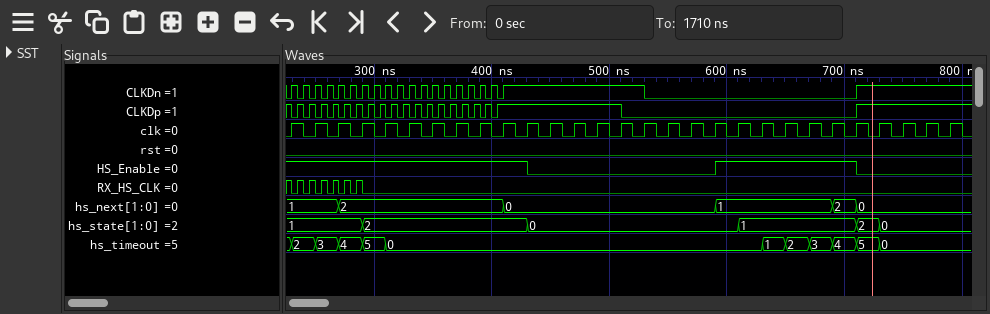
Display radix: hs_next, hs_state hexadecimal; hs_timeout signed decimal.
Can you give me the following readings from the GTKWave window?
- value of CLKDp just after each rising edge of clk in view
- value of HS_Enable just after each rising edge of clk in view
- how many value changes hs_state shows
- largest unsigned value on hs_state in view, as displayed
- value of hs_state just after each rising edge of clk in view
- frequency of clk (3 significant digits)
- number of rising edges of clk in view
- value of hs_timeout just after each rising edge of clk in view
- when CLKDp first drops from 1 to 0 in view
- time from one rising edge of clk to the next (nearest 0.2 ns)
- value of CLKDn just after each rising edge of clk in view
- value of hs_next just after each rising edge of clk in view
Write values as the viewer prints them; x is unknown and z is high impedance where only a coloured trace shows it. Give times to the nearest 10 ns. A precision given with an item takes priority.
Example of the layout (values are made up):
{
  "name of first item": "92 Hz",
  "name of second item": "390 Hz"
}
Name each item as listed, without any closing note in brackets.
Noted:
{
  "value of CLKDp just after each rising edge of clk in view": "0 0 0 0 0 0 0 0 0 1 1 1 1 1 0 0 0 0 0 0 0 0 0 0 1 1 1 1 1",
  "value of HS_Enable just after each rising edge of clk in view": "1 1 1 1 1 1 1 1 1 1 0 0 0 0 0 0 0 0 1 1 1 1 1 1 0 0 0 0 0",
  "how many value changes hs_state shows": "5",
  "largest unsigned value on hs_state in view, as displayed": "2",
  "value of hs_state just after each rising edge of clk in view": "1, 1, 1, 2, 2, 2, 2, 2, 2, 2, 0, 0, 0, 0, 0, 0, 0, 0, 0, 1, 1, 1, 1, 1, 2, 0, 0, 0, 0",
  "frequency of clk": "50.0 MHz",
  "number of rising edges of clk in view": "29",
  "value of hs_timeout just after each rising edge of clk in view": "2, 3, 4, 5, 0, 0, 0, 0, 0, 0, 0, 0, 0, 0, 0, 0, 0, 0, 0, 0, 1, 2, 3, 4, 5, 0, 0, 0, 0",
  "when CLKDp first drops from 1 to 0 in view": "230 ns",
  "time from one rising edge of clk to the next": "20 ns",
  "value of CLKDn just after each rising edge of clk in view": "1 1 1 1 1 1 1 1 1 1 1 1 1 1 1 0 0 0 0 0 0 0 0 0 1 1 1 1 1",
  "value of hs_next just after each rising edge of clk in view": "1, 1, 2, 2, 2, 2, 2, 2, 2, 0, 0, 0, 0, 0, 0, 0, 0, 0, 1, 1, 1, 1, 1, 2, 0, 0, 0, 0, 0"
}
